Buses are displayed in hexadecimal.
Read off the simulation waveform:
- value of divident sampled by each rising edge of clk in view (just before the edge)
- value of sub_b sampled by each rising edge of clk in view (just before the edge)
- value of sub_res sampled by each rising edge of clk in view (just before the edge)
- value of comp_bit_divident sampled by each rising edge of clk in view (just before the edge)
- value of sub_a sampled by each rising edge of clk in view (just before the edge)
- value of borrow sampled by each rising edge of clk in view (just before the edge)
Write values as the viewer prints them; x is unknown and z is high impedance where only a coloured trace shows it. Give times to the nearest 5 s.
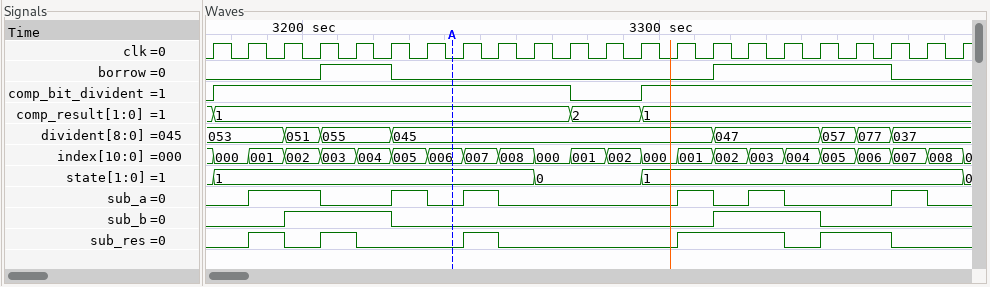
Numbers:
053, 053, 053, 051, 055, 055, 045, 045, 045, 045, 045, 045, 045, 045, 045, 047, 047, 047, 057, 077, 037, 037
0 0 0 1 1 1 0 0 0 0 0 0 0 0 0 1 1 1 0 0 0 0
0 0 1 0 1 0 0 0 1 0 0 0 0 0 1 1 1 0 1 1 0 0
0 1 1 1 1 1 1 1 1 1 1 0 0 1 1 1 1 1 1 1 1 1
0 0 1 1 0 0 1 0 1 0 0 0 0 0 1 0 1 0 0 0 1 0
0 0 0 0 1 1 0 0 0 0 0 0 0 0 0 1 1 1 1 1 0 0
